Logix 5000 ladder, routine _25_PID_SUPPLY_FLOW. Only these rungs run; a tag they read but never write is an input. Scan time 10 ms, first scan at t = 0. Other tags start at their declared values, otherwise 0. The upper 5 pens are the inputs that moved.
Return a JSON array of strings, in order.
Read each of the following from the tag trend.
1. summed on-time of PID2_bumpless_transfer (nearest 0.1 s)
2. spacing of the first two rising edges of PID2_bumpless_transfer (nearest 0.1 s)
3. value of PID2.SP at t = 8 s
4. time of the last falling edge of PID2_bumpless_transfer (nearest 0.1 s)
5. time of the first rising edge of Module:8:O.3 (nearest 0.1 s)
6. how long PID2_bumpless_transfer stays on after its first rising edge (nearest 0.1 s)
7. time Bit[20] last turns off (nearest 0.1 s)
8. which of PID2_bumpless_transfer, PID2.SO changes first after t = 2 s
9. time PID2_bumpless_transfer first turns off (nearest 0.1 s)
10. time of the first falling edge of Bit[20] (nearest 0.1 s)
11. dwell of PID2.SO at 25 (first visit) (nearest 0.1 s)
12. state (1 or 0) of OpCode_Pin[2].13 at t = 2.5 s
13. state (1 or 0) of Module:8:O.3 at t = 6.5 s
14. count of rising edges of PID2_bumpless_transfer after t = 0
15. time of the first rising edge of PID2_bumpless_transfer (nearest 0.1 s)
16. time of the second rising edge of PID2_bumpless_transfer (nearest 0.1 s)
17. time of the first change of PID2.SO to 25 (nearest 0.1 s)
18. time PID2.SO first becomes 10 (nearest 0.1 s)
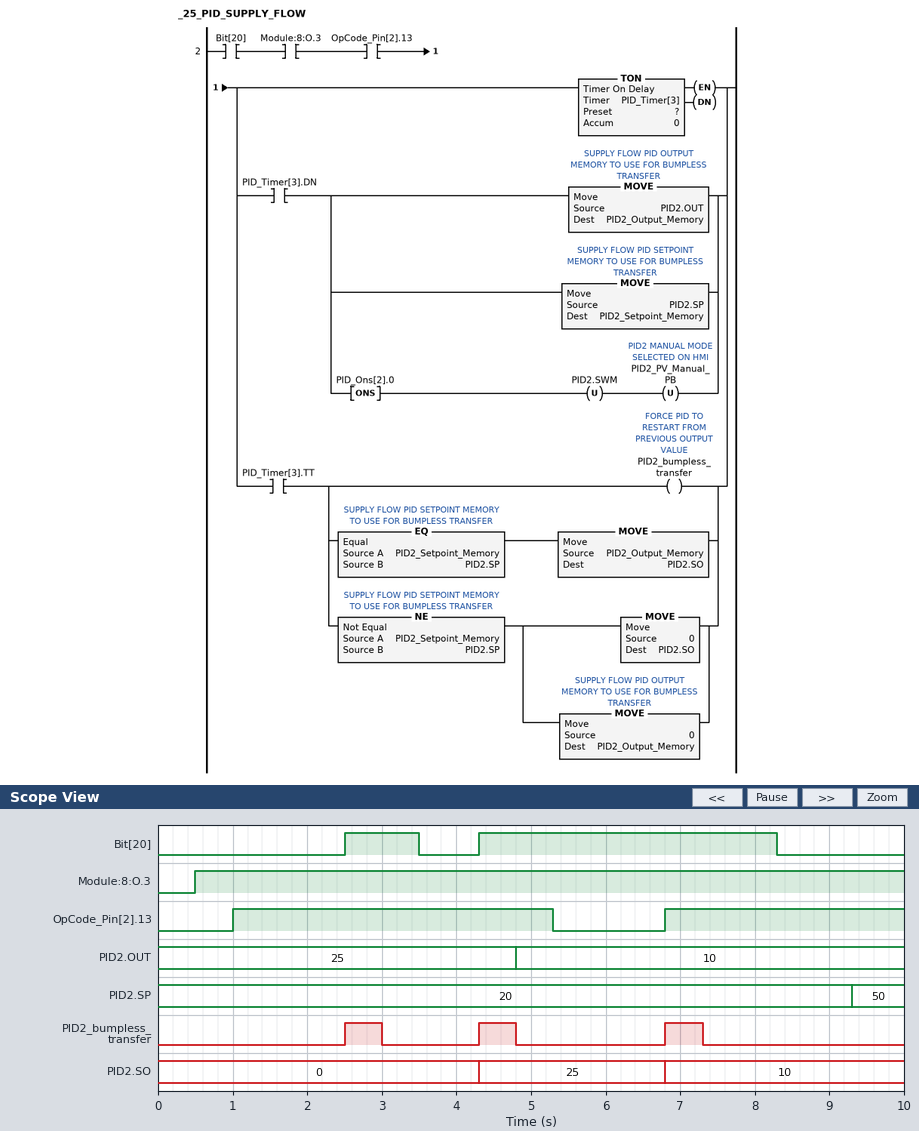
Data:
["1.5 s", "1.8 s", "20", "7.3 s", "0.5 s", "0.5 s", "8.3 s", "PID2_bumpless_transfer", "3.0 s", "3.5 s", "2.5 s", "1", "1", "3", "2.5 s", "4.3 s", "4.3 s", "6.8 s"]
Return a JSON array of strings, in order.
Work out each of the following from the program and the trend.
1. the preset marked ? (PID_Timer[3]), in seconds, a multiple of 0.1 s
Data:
["0.5 s"]
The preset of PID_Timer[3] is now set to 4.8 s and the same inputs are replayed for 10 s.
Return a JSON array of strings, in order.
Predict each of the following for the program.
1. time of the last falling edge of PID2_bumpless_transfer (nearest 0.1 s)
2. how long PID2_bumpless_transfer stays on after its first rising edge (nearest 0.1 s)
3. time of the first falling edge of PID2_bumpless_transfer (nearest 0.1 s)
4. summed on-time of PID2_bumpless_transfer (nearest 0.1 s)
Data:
["8.3 s", "1.0 s", "3.5 s", "3.5 s"]
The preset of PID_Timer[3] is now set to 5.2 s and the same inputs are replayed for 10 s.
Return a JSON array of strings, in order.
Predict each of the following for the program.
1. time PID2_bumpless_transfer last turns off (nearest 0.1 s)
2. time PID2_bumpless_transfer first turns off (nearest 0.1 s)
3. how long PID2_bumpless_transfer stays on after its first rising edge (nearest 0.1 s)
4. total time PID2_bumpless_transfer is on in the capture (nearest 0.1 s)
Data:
["8.3 s", "3.5 s", "1.0 s", "3.5 s"]
